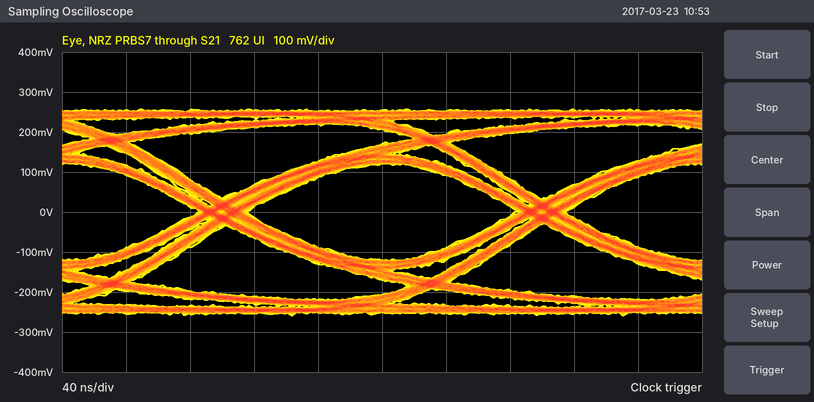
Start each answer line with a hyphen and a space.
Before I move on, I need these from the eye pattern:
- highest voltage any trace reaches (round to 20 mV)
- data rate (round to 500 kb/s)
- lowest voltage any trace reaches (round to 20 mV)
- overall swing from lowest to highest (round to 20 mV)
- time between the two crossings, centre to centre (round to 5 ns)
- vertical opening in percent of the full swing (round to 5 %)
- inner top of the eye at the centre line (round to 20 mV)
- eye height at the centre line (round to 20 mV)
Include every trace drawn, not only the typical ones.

- 260 mV
- 5.0 Mb/s
- -260 mV
- 520 mV
- 200 ns
- 45 %
- 120 mV
- 240 mV
